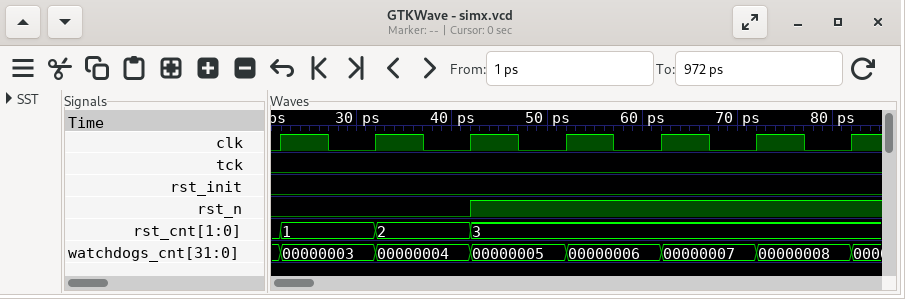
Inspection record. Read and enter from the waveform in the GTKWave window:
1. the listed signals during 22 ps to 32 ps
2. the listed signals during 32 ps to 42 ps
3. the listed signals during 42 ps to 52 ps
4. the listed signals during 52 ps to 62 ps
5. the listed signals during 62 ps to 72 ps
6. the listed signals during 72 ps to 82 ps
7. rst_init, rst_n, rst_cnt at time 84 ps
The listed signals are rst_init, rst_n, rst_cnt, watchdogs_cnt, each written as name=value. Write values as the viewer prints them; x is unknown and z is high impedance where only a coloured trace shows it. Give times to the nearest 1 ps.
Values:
rst_init=0, rst_n=0, rst_cnt=1, watchdogs_cnt=00000003
rst_init=0, rst_n=0, rst_cnt=2, watchdogs_cnt=00000004
rst_init=0, rst_n=1, rst_cnt=3, watchdogs_cnt=00000005
rst_init=0, rst_n=1, rst_cnt=3, watchdogs_cnt=00000006
rst_init=0, rst_n=1, rst_cnt=3, watchdogs_cnt=00000007
rst_init=0, rst_n=1, rst_cnt=3, watchdogs_cnt=00000008
rst_init=0, rst_n=1, rst_cnt=3
